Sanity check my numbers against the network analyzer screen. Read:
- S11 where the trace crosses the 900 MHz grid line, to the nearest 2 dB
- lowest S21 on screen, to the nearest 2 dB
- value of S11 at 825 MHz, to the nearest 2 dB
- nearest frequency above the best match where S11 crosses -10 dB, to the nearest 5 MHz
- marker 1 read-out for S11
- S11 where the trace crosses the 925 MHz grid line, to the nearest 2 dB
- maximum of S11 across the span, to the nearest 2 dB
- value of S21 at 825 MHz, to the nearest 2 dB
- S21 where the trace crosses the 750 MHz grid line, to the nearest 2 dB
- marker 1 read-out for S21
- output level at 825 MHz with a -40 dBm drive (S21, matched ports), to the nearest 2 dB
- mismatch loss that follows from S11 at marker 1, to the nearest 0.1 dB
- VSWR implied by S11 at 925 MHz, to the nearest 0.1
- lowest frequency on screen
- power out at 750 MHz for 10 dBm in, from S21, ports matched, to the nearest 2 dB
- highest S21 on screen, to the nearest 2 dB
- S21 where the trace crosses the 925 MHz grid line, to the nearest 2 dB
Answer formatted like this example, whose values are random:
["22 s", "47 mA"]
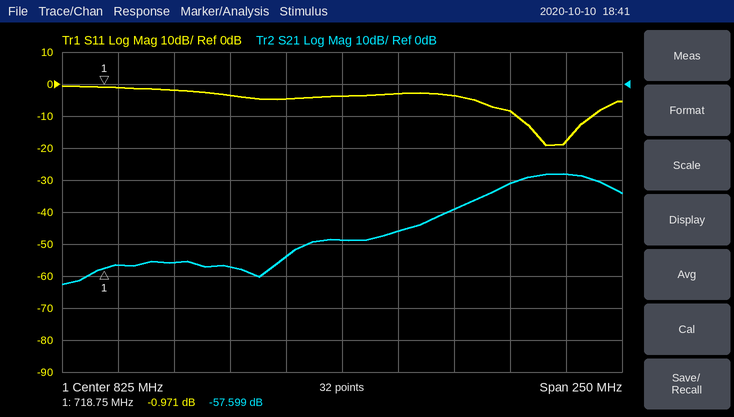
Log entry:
["-8 dB", "-62 dB", "-4 dB", "935 MHz", "-0.971 dB", "-18 dB", "0 dB", "-48 dB", "-56 dB", "-57.599 dB", "-88 dBm", "7.0 dB", "1.3", "700 MHz", "-46 dBm", "-28 dB", "-28 dB"]
